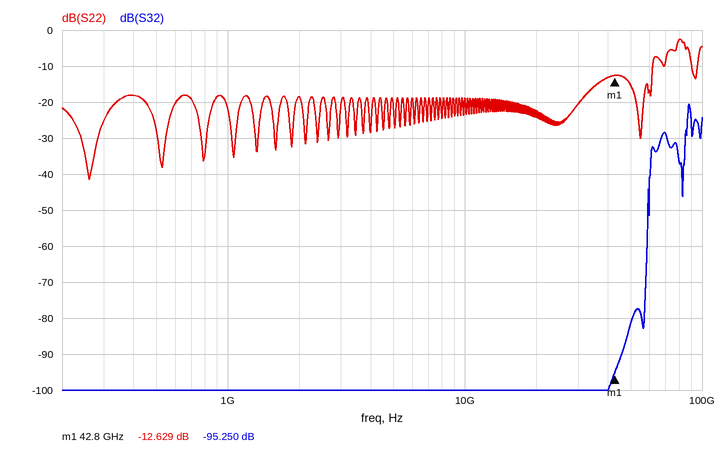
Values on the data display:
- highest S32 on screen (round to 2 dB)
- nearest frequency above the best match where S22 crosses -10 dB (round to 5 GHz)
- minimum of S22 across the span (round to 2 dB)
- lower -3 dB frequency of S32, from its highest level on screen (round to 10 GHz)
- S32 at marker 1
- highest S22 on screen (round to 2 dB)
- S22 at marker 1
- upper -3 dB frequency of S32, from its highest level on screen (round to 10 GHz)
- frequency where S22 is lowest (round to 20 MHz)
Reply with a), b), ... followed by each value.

a) -20 dB
b) 60 GHz
c) -42 dB
d) 90 GHz
e) -95.250 dB
f) -2 dB
g) -12.629 dB
h) 90 GHz
i) 260 MHz
